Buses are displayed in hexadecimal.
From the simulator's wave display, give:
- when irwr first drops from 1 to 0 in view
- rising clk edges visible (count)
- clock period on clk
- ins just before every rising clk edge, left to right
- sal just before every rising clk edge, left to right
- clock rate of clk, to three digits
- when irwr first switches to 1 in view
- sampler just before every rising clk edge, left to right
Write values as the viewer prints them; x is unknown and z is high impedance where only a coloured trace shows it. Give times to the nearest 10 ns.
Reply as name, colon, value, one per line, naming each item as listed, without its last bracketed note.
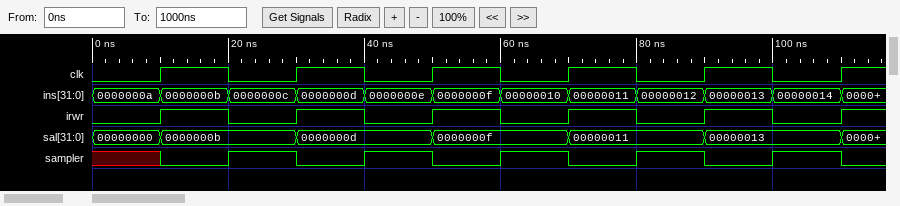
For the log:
when irwr first drops from 1 to 0 in view: 20 ns
rising clk edges visible: 6
clock period on clk: 20 ns
ins just before every rising clk edge, left to right: 0000000a, 0000000c, 0000000e, 00000010, 00000012, 00000014
sal just before every rising clk edge, left to right: 00000000, 0000000b, 0000000d, 0000000f, 00000011, 00000013
clock rate of clk, to three digits: 50.0 MHz
when irwr first switches to 1 in view: 10 ns
sampler just before every rising clk edge, left to right: x 1 1 1 1 1
